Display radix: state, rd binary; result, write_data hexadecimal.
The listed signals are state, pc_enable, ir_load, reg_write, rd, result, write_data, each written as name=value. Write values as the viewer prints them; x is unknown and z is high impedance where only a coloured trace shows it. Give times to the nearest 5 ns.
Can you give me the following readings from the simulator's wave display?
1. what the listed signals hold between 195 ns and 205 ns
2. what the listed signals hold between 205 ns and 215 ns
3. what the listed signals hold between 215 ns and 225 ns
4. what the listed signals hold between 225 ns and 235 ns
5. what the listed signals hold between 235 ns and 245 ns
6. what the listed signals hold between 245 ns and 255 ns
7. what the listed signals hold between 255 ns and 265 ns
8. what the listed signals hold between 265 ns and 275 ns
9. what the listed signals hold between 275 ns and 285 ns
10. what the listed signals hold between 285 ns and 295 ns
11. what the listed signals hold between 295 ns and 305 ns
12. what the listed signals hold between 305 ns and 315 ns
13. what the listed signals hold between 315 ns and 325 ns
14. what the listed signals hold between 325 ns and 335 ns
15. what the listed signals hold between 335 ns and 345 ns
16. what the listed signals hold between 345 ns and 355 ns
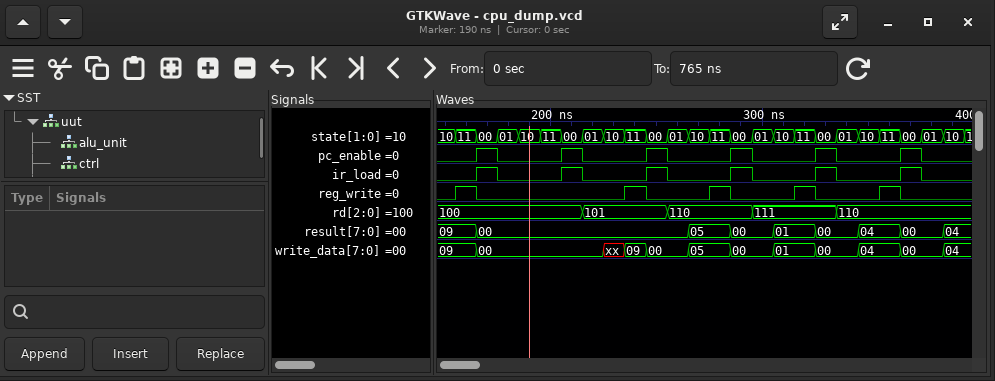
state=11, pc_enable=0, ir_load=0, reg_write=0, rd=100, result=00, write_data=00
state=00, pc_enable=1, ir_load=1, reg_write=0, rd=100, result=00, write_data=00
state=01, pc_enable=0, ir_load=0, reg_write=0, rd=101, result=00, write_data=00
state=10, pc_enable=0, ir_load=0, reg_write=0, rd=101, result=00, write_data=xx
state=11, pc_enable=0, ir_load=0, reg_write=1, rd=101, result=00, write_data=09
state=00, pc_enable=1, ir_load=1, reg_write=0, rd=101, result=00, write_data=00
state=01, pc_enable=0, ir_load=0, reg_write=0, rd=110, result=00, write_data=00
state=10, pc_enable=0, ir_load=0, reg_write=0, rd=110, result=05, write_data=05
state=11, pc_enable=0, ir_load=0, reg_write=1, rd=110, result=05, write_data=05
state=00, pc_enable=1, ir_load=1, reg_write=0, rd=110, result=00, write_data=00
state=01, pc_enable=0, ir_load=0, reg_write=0, rd=111, result=00, write_data=00
state=10, pc_enable=0, ir_load=0, reg_write=0, rd=111, result=01, write_data=01
state=11, pc_enable=0, ir_load=0, reg_write=1, rd=111, result=01, write_data=01
state=00, pc_enable=1, ir_load=1, reg_write=0, rd=111, result=00, write_data=00
state=01, pc_enable=0, ir_load=0, reg_write=0, rd=110, result=00, write_data=00
state=10, pc_enable=0, ir_load=0, reg_write=0, rd=110, result=04, write_data=04
